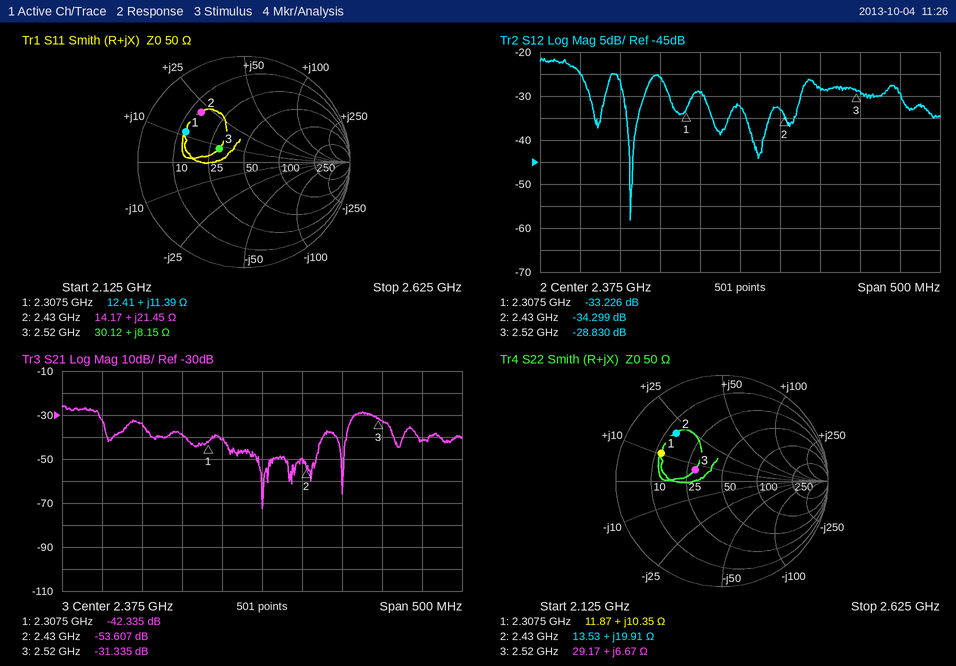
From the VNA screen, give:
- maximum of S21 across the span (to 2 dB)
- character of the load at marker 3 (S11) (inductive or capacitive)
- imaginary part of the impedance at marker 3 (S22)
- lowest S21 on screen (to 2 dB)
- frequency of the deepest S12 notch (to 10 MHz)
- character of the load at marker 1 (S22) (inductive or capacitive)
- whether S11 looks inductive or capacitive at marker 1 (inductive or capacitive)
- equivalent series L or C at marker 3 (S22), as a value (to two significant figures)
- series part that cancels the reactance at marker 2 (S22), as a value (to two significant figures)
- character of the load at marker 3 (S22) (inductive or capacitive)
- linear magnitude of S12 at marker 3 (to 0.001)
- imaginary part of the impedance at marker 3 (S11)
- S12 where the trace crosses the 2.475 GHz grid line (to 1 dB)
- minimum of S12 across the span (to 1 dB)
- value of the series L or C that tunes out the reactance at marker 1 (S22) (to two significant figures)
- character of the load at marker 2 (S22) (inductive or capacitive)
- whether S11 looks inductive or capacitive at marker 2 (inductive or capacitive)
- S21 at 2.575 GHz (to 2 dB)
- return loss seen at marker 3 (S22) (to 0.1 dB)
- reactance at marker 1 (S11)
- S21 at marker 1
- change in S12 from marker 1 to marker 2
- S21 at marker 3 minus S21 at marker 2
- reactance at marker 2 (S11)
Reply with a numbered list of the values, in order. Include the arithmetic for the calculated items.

1. -26 dB
2. inductive
3. +6.67 Ω
4. -72 dB
5. 2.24 GHz
6. inductive
7. inductive
8. L = 6.67 Ω/(2π × 2.52 GHz) ≈ 421 pH, so 420 pH to two significant figures
9. C = 1/(2π × 2.43 GHz × 19.91 Ω) ≈ 3.3 pF
10. inductive
11. 10^(-28.83/20) ≈ 0.036
12. +8.15 Ω
13. -28 dB
14. -58 dB
15. C = 1/(2π × 2.3075 GHz × 10.35 Ω) ≈ 6.7 pF
16. inductive
17. inductive
18. -42 dB
19. 11.2 dB
20. +11.39 Ω
21. -42.335 dB
22. -34.299 − (-33.226) = -1.073 dB
23. -31.335 − (-53.607) = 22.272 dB
24. +21.45 Ω
